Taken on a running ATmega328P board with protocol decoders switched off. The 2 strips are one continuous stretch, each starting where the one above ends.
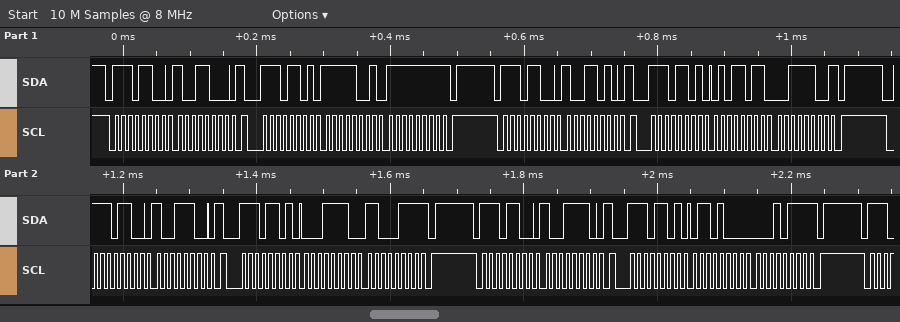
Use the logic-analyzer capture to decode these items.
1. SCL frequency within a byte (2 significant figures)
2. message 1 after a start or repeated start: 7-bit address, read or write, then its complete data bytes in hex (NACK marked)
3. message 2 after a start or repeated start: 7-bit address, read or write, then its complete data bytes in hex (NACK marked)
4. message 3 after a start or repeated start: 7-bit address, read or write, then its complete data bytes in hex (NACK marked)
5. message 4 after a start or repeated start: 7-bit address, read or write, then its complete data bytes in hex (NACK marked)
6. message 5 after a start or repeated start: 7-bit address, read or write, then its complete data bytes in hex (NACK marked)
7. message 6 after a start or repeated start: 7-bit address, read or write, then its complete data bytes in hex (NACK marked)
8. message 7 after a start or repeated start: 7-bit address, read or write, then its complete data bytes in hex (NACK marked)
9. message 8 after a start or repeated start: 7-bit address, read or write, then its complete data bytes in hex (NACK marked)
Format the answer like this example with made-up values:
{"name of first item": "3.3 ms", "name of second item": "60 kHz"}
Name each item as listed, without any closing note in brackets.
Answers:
{"SCL frequency within a byte": "100 kHz", "message 1 after a start or repeated start: 7-bit address, read or write, then its complete data bytes in hex": "0x76 write: 98", "message 2 after a start or repeated start: 7-bit address, read or write, then its complete data bytes in hex": "0x76 read: F9 FF NACK", "message 3 after a start or repeated start: 7-bit address, read or write, then its complete data bytes in hex": "0x76 write: 9A", "message 4 after a start or repeated start: 7-bit address, read or write, then its complete data bytes in hex": "0x76 read: 5B 3C NACK", "message 5 after a start or repeated start: 7-bit address, read or write, then its complete data bytes in hex": "0x76 write: 9C", "message 6 after a start or repeated start: 7-bit address, read or write, then its complete data bytes in hex": "0x76 read: 1E C7 NACK", "message 7 after a start or repeated start: 7-bit address, read or write, then its complete data bytes in hex": "0x76 write: 9E", "message 8 after a start or repeated start: 7-bit address, read or write, then its complete data bytes in hex": "0x76 read: 68 17 NACK"}
